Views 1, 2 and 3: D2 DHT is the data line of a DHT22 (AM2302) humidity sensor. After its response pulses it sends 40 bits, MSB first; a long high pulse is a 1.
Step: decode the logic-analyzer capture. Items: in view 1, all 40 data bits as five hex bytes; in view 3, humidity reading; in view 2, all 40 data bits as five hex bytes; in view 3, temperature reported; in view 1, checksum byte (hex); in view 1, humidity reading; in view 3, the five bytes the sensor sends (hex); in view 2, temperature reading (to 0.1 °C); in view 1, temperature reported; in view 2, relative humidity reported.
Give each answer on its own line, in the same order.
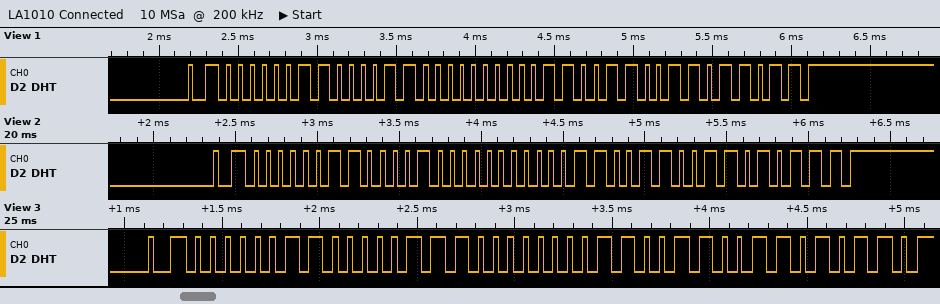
03 0C 00 CC DB
77.5 %
03 08 00 CC D7
20.4 °C
0xDB
78.0 %
03 07 00 CC D6
20.4 °C
20.4 °C
77.6 %
